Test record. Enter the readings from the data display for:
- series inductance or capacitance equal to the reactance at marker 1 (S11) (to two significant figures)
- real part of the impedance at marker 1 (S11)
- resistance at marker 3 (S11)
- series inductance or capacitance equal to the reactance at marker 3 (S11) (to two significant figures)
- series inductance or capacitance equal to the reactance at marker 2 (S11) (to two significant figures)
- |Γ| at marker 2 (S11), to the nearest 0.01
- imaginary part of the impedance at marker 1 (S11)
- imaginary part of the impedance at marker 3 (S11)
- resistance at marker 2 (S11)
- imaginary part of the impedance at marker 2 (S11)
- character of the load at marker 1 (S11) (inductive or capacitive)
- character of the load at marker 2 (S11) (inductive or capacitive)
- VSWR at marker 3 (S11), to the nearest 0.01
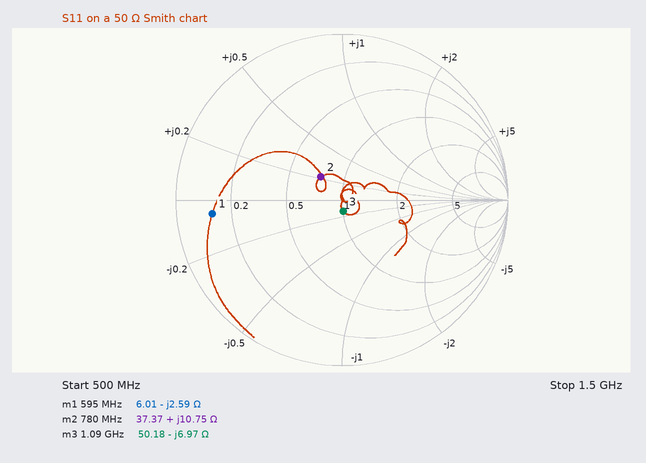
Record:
100 pF
6.01 Ω
50.18 Ω
21 pF
2.2 nH
0.19
-2.59 Ω
-6.97 Ω
37.37 Ω
+10.75 Ω
capacitive
inductive
1.15
